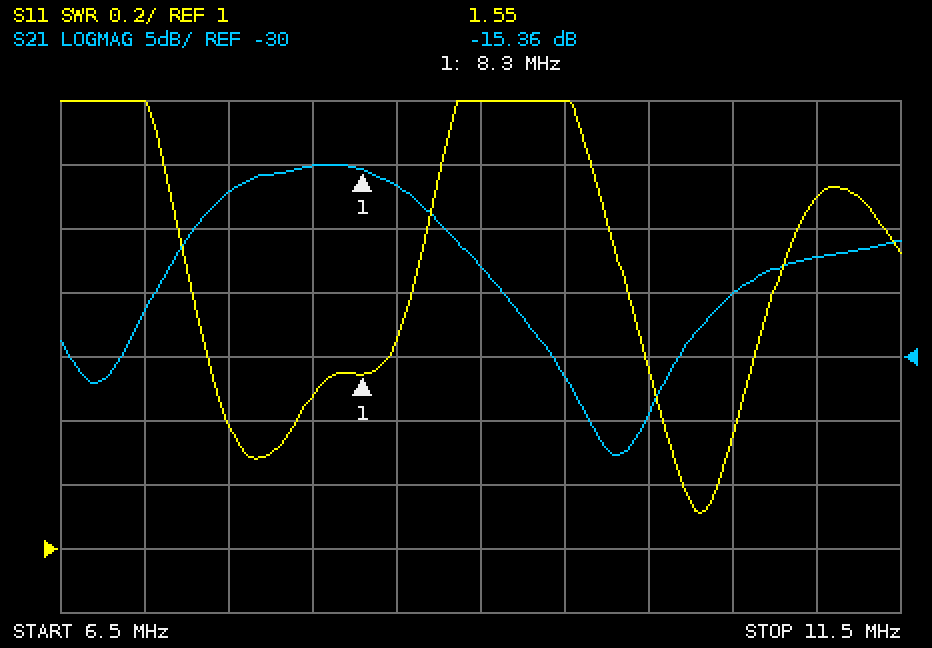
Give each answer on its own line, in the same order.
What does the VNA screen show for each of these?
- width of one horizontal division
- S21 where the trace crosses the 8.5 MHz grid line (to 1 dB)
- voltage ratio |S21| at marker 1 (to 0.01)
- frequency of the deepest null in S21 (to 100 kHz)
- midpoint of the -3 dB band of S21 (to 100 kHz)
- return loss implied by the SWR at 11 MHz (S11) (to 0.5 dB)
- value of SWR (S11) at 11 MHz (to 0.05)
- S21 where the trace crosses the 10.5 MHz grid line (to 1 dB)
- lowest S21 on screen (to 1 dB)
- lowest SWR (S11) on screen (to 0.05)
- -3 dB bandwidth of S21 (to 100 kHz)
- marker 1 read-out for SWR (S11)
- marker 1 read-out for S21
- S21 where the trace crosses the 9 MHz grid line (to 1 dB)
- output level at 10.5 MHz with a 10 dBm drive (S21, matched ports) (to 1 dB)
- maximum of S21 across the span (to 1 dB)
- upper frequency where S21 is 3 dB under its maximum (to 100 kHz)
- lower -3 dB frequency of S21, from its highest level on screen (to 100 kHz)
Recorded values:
500 kHz
-17 dB
0.17
9.8 MHz
8.0 MHz
9.0 dB
2.10
-25 dB
-38 dB
1.10
1.2 MHz
1.55
-15.36 dB
-23 dB
-15 dBm
-15 dB
8.6 MHz
7.4 MHz
